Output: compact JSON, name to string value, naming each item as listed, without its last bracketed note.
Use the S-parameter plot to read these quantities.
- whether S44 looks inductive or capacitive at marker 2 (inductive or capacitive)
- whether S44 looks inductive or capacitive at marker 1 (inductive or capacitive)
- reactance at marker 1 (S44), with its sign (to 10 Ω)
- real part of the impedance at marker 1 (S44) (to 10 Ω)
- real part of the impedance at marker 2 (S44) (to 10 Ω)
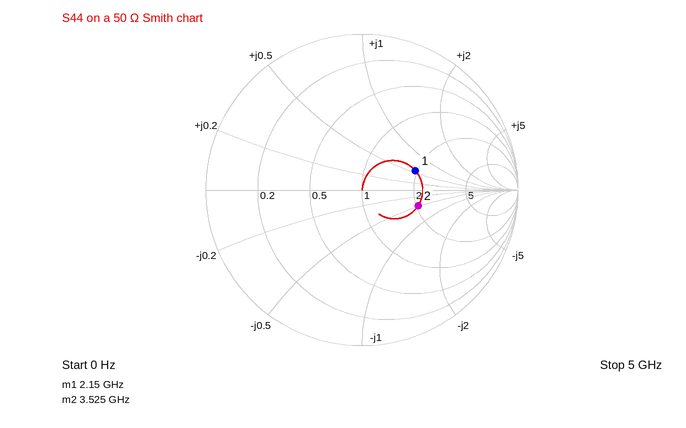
{"whether S44 looks inductive or capacitive at marker 2": "capacitive", "whether S44 looks inductive or capacitive at marker 1": "inductive", "reactance at marker 1 (S44), with its sign": "+30 Ω", "real part of the impedance at marker 1 (S44)": "100 Ω", "real part of the impedance at marker 2 (S44)": "100 Ω"}
